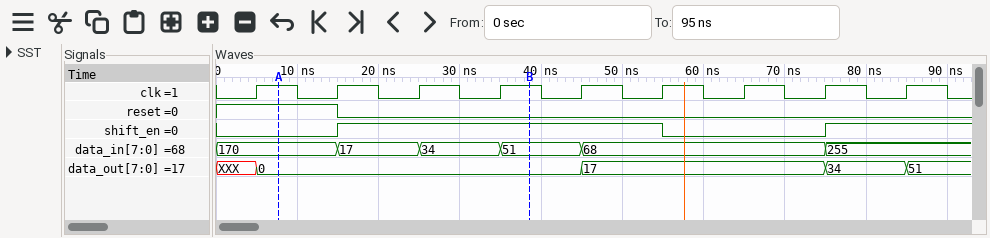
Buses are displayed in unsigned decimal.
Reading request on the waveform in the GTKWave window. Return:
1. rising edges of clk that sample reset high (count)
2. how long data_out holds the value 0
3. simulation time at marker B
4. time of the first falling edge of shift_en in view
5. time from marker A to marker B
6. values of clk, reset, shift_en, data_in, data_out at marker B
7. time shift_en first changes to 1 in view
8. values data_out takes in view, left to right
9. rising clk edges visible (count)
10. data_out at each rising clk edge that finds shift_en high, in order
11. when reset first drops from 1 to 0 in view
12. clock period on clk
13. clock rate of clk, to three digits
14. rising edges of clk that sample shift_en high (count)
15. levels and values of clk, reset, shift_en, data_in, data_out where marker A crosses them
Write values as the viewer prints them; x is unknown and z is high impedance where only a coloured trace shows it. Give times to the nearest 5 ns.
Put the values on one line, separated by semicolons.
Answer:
2; 40 ns; 40 ns; 55 ns; 30 ns; clk=1, reset=0, shift_en=1, data_in=51, data_out=0; 15 ns; XXX, 0, 17, 34, 51; 9; 0, 0, 0, 17, 34; 15 ns; 10 ns; 100 MHz; 5; clk=1, reset=1, shift_en=0, data_in=170, data_out=0
